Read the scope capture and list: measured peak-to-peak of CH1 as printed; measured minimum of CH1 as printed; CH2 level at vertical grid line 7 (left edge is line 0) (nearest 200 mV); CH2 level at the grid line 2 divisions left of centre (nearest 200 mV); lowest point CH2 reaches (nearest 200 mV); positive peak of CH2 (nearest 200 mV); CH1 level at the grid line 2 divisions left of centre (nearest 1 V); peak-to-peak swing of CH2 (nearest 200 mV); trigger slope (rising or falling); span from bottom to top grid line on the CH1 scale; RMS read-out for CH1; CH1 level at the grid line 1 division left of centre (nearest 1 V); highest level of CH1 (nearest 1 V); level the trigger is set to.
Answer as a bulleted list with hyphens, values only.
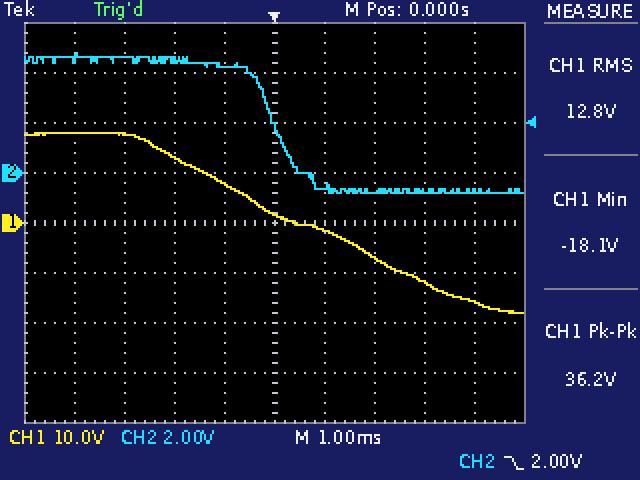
- 36.2 V
- -18.1 V
- -800 mV
- 4.6 V
- -800 mV
- 4.8 V
- 13 V
- 5.6 V
- falling
- 80 V
- 12.8 V
- 8 V
- 18 V
- 2.00 V
